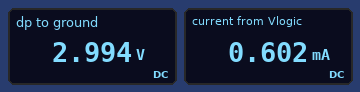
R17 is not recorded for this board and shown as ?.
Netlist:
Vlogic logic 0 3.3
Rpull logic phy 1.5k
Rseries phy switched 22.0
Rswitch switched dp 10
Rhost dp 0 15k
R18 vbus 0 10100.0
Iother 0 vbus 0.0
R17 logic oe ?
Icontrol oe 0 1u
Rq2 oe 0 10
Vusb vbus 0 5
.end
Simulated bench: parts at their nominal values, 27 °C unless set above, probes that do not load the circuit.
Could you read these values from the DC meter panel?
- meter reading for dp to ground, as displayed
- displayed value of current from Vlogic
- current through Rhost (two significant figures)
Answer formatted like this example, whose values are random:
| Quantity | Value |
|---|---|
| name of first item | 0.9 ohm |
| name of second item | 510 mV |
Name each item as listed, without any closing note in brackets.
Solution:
| Quantity | Value |
|---|---|
| meter reading for dp to ground, as displayed | 2.994 V |
| displayed value of current from Vlogic | 0.602 mA |
| current through Rhost | 200 µA |
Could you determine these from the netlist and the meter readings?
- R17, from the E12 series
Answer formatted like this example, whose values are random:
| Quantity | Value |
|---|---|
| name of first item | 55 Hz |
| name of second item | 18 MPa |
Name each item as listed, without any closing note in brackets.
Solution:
| Quantity | Value |
|---|---|
| R17, from the E12 series | 8.2 kΩ |
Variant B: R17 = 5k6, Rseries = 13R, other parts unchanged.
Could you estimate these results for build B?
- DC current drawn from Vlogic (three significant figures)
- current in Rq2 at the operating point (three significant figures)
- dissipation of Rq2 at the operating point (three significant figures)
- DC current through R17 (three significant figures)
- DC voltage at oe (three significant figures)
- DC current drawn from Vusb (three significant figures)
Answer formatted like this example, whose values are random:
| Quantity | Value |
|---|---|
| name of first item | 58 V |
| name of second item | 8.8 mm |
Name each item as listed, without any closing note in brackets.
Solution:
| Quantity | Value |
|---|---|
| DC current drawn from Vlogic | 788 µA |
| current in Rq2 at the operating point | 587 µA |
| dissipation of Rq2 at the operating point | 3.45 µW |
| DC current through R17 | 588 µA |
| DC voltage at oe | 5.87 mV |
| DC current drawn from Vusb | 495 µA |
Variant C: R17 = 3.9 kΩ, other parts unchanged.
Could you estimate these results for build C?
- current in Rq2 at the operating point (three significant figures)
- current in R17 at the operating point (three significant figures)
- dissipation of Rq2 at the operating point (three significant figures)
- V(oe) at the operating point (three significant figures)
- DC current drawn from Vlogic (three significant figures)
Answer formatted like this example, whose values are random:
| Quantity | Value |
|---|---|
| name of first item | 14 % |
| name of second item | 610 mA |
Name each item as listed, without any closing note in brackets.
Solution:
| Quantity | Value |
|---|---|
| current in Rq2 at the operating point | 843 µA |
| current in R17 at the operating point | 844 µA |
| dissipation of Rq2 at the operating point | 7.11 µW |
| V(oe) at the operating point | 8.43 mV |
| DC current drawn from Vlogic | 1.04 mA |
